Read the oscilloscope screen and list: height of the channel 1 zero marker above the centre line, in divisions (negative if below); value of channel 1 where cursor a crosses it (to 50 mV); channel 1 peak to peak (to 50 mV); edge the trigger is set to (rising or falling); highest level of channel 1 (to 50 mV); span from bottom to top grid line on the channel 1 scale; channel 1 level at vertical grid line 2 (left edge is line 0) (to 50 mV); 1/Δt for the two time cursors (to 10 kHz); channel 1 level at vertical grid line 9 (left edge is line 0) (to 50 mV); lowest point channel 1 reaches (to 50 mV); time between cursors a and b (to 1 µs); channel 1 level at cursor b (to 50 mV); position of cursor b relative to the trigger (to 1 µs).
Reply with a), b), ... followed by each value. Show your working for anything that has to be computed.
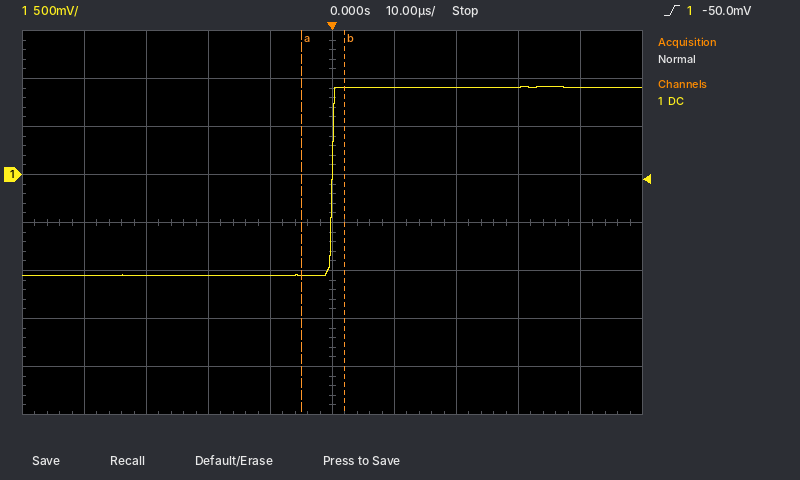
a) +1.0 div
b) -1.05 V
c) 900 mV − (-1.05 V) = 1.95 V
d) rising
e) 900 mV
f) 4 V
g) -1.05 V
h) 1 / 7 µs ≈ 140 kHz
i) 900 mV
j) -1.05 V
k) 7 µs
l) 900 mV
m) +2 µs
